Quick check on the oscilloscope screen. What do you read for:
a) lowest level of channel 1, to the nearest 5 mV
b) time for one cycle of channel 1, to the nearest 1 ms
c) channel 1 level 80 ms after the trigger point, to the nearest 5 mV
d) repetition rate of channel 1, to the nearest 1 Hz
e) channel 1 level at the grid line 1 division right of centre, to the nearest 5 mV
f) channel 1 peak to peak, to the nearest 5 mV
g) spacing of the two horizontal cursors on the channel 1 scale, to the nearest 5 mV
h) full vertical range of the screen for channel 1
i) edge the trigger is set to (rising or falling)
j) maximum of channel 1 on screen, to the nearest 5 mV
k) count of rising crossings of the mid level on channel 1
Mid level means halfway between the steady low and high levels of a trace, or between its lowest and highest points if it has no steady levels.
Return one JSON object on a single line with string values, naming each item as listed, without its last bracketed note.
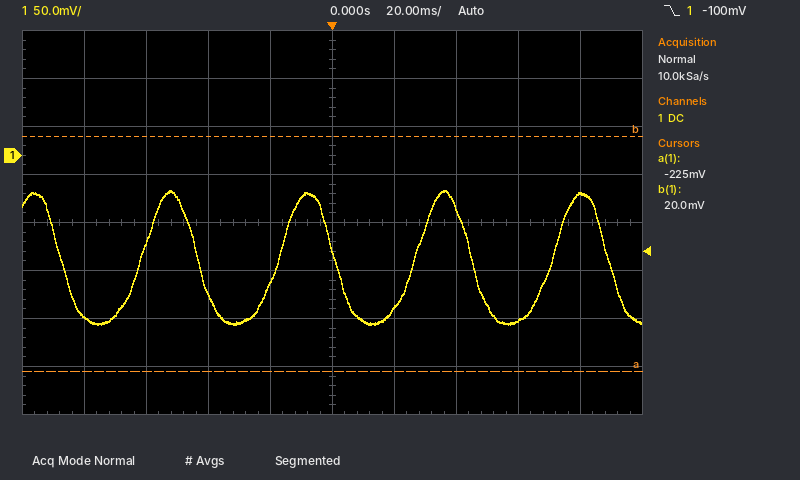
{"lowest level of channel 1, to the nearest 5 mV": "-175 mV", "time for one cycle of channel 1, to the nearest 1 ms": "44 ms", "channel 1 level 80 ms after the trigger point, to the nearest 5 mV": "-40 mV", "repetition rate of channel 1, to the nearest 1 Hz": "23 Hz", "channel 1 level at the grid line 1 division right of centre, to the nearest 5 mV": "-160 mV", "channel 1 peak to peak, to the nearest 5 mV": "140 mV", "spacing of the two horizontal cursors on the channel 1 scale, to the nearest 5 mV": "245 mV", "full vertical range of the screen for channel 1": "400 mV", "edge the trigger is set to": "falling", "maximum of channel 1 on screen, to the nearest 5 mV": "-35 mV", "count of rising crossings of the mid level on channel 1": "4"}
